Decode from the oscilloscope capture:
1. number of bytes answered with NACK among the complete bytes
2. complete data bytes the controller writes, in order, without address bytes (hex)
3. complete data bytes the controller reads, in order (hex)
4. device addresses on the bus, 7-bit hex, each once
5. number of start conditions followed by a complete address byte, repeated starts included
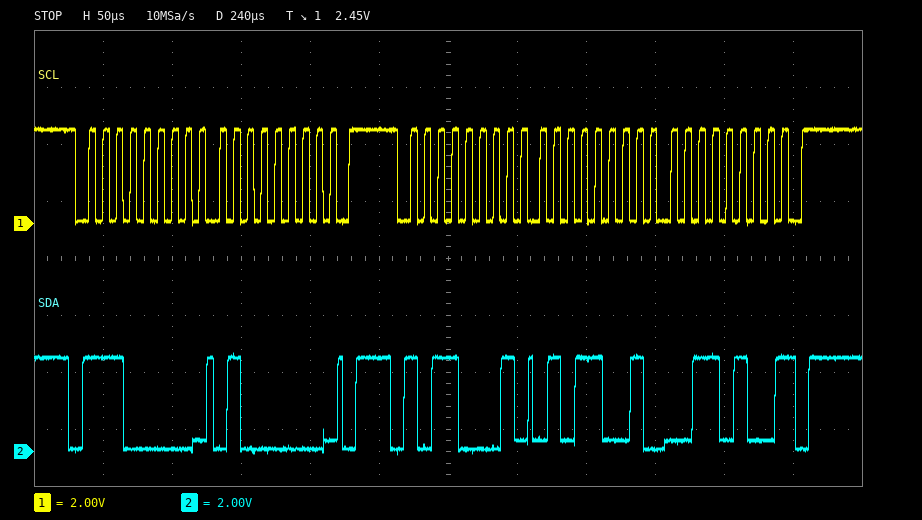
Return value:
1
40
59 34
0x70 0x58
2
